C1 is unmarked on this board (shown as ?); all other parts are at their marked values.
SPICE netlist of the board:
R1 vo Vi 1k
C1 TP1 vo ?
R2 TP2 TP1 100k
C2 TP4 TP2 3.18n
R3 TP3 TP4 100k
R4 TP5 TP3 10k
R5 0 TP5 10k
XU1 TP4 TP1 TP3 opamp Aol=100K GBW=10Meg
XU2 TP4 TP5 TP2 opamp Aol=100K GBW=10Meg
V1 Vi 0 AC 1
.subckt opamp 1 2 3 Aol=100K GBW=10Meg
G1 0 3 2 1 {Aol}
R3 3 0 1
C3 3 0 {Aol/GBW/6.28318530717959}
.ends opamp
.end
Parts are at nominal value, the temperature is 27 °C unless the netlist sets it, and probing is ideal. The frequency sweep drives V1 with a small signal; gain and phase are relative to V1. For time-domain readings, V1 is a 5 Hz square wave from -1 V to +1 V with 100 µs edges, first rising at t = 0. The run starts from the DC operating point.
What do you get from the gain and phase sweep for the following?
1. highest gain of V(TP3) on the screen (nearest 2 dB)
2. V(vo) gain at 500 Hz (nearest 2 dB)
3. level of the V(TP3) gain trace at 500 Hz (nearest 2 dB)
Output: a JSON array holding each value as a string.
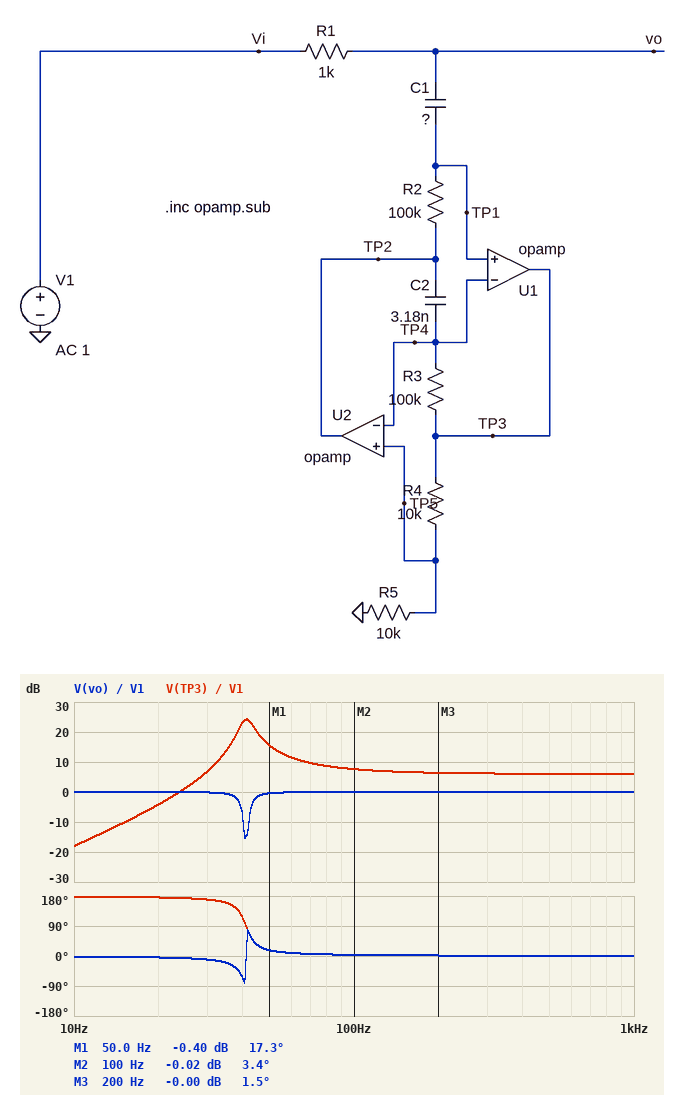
["24 dB", "0 dB", "6 dB"]
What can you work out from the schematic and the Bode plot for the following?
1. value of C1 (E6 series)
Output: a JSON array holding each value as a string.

["470 nF"]
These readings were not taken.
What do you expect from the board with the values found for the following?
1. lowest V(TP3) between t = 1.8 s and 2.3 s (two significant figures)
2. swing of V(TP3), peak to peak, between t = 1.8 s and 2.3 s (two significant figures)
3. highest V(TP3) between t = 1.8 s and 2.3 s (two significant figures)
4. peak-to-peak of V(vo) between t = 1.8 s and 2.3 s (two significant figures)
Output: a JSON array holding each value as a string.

["-3.4 V", "6.8 V", "3.4 V", "2.3 V"]
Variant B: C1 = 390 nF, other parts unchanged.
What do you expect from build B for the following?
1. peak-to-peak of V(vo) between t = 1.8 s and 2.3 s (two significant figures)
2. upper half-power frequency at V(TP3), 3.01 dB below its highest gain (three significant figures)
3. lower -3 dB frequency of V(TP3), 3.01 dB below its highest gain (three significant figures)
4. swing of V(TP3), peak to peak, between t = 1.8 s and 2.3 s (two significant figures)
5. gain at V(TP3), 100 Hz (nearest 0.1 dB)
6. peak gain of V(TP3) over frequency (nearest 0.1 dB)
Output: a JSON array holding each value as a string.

["2.4 V", "48.1 Hz", "43.0 Hz", "10 V", "8.0 dB", "25.1 dB"]
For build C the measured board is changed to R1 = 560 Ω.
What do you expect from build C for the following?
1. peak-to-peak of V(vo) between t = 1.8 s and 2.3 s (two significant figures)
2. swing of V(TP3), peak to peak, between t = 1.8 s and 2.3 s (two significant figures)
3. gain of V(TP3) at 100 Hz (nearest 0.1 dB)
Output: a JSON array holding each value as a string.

["2.2 V", "5.9 V", "7.6 dB"]
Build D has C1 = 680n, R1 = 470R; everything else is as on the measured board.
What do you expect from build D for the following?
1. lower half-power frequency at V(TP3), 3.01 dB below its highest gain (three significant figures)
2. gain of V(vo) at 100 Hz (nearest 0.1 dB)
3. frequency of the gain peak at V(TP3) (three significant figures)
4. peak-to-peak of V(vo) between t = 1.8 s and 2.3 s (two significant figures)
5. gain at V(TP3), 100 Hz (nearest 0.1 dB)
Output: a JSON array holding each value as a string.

["33.1 Hz", "0 dB", "34.3 Hz", "2.4 V", "7.1 dB"]
